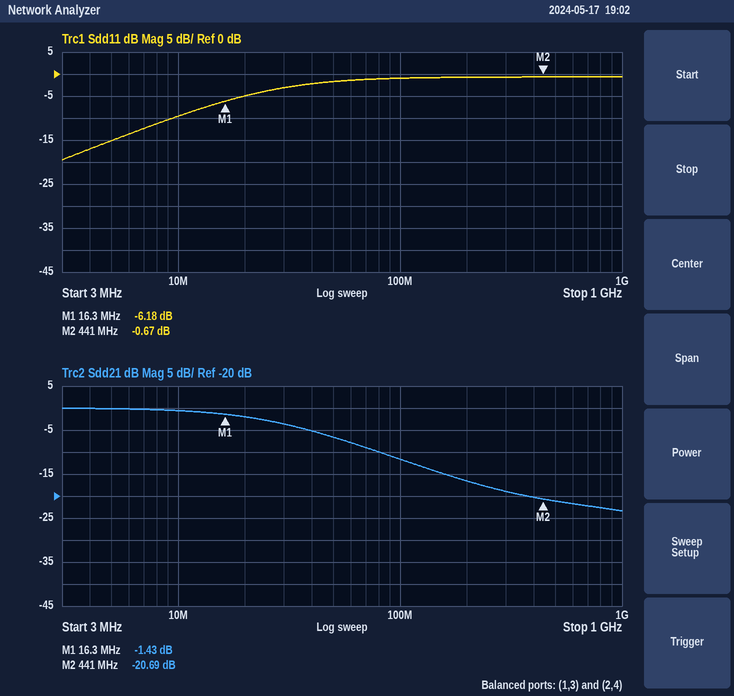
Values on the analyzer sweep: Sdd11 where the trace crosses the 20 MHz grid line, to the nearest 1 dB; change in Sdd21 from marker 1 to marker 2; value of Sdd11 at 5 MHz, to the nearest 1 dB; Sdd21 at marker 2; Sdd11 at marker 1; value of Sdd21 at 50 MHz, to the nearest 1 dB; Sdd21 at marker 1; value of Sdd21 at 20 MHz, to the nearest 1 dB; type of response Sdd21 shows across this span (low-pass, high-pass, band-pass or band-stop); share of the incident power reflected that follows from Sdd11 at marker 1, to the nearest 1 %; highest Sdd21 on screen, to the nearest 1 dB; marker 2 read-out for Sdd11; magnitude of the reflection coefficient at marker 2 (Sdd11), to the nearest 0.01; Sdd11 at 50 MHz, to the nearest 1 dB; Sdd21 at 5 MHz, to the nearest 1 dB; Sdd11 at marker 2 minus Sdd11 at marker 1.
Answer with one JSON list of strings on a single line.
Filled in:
["-5 dB", "-19.26 dB", "-15 dB", "-20.69 dB", "-6.18 dB", "-7 dB", "-1.43 dB", "-2 dB", "low-pass", "24 %", "0 dB", "-0.67 dB", "0.93", "-2 dB", "0 dB", "5.51 dB"]
